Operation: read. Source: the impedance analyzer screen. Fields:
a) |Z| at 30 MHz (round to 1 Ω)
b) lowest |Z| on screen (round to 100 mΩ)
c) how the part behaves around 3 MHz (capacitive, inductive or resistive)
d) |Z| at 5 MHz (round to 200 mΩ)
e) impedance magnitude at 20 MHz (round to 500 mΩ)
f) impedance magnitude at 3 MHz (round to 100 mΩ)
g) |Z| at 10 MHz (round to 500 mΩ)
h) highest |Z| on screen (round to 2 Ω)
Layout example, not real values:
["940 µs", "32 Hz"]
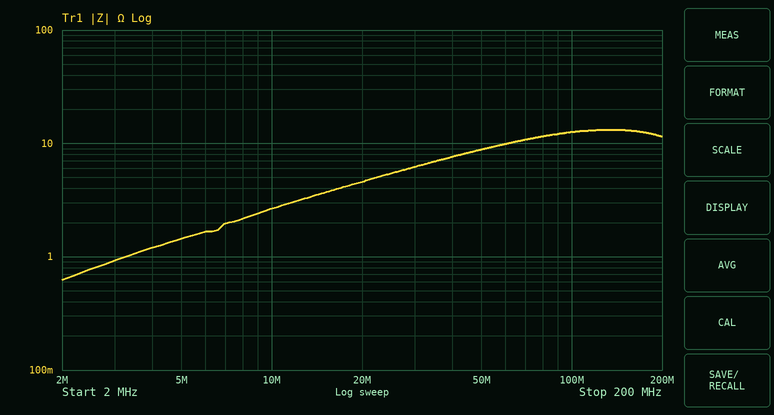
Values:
["6 Ω", "600 mΩ", "inductive", "1.4 Ω", "4.5 Ω", "900 mΩ", "2.5 Ω", "14 Ω"]
